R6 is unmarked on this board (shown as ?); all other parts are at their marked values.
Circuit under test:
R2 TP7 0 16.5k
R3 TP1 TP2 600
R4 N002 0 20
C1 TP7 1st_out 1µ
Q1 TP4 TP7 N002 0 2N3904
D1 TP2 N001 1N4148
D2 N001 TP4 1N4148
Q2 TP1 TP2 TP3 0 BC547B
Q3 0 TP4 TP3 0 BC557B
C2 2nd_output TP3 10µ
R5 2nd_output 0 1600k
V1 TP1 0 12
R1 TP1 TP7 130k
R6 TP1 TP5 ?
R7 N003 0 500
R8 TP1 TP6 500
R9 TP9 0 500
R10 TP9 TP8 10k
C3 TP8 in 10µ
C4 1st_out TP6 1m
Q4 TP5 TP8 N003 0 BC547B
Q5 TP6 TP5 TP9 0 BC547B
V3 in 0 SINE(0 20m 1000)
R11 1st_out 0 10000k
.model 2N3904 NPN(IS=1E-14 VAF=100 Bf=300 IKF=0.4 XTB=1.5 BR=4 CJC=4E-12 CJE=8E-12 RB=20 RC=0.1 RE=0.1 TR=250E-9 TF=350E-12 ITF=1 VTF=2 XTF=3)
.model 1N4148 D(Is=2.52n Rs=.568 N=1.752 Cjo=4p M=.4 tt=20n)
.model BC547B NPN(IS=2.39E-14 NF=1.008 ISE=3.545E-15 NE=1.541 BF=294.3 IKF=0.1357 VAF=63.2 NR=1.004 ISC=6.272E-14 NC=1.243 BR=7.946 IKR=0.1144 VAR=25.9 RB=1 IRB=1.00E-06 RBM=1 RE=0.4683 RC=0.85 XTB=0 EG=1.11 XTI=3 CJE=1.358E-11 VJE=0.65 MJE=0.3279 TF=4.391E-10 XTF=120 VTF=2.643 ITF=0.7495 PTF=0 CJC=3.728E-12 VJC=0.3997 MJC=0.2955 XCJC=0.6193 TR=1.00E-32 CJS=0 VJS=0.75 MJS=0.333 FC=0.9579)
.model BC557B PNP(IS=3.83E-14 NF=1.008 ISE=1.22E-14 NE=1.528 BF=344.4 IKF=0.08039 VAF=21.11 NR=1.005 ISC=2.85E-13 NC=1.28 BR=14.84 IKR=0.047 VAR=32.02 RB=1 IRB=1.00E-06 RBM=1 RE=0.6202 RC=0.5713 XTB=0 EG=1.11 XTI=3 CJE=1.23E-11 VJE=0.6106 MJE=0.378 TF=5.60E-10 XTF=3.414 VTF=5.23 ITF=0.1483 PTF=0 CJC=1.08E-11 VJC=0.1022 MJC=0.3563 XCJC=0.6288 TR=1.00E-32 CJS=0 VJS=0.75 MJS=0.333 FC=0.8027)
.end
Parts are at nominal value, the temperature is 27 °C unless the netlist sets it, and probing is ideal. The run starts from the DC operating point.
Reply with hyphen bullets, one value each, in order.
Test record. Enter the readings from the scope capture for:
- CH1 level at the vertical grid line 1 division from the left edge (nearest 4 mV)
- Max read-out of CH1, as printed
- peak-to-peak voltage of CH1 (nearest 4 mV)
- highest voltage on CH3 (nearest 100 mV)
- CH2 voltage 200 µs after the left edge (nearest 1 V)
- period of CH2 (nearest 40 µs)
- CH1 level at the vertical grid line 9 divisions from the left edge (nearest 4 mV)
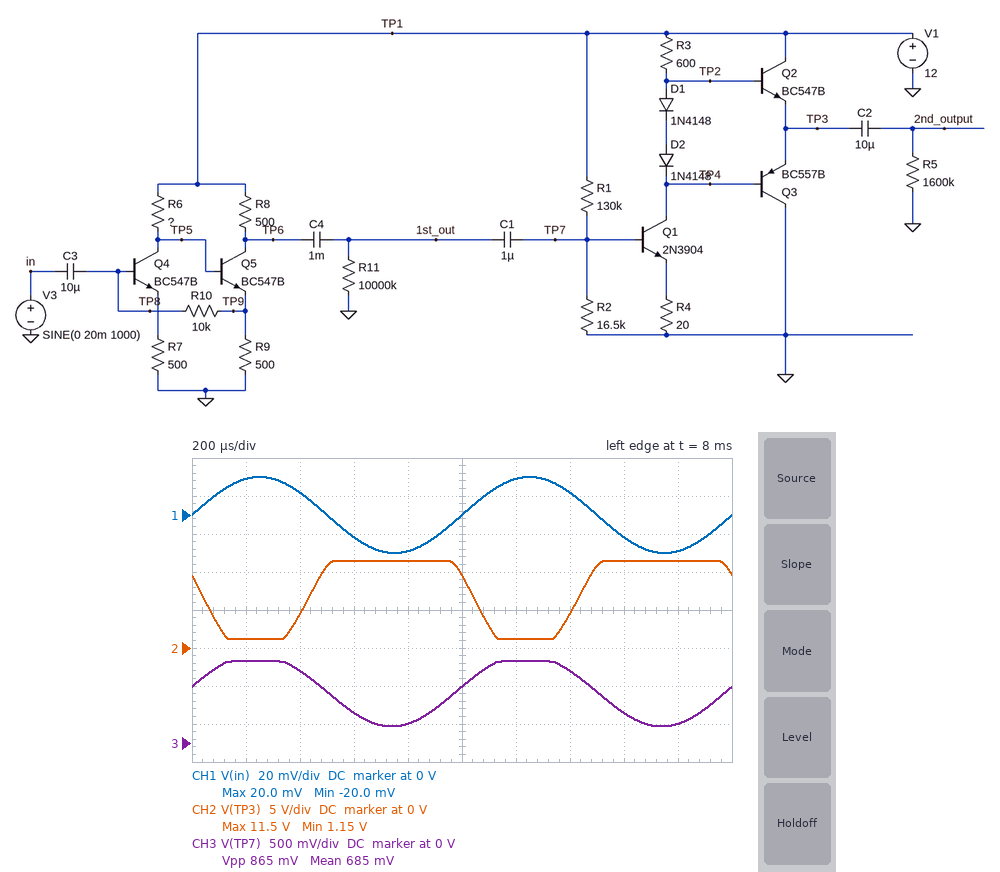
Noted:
- 20 mV
- 20.0 mV
- 40 mV
- 1.1 V
- 1 V
- 1.00 ms
- -20 mV
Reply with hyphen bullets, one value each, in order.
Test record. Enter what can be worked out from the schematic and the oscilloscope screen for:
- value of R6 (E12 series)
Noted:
- 15 kΩ
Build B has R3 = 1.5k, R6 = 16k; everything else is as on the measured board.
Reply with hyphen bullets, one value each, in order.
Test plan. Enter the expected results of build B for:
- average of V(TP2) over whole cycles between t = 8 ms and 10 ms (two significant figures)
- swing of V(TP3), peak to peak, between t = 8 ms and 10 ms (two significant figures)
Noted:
- 8.4 V
- 11 V
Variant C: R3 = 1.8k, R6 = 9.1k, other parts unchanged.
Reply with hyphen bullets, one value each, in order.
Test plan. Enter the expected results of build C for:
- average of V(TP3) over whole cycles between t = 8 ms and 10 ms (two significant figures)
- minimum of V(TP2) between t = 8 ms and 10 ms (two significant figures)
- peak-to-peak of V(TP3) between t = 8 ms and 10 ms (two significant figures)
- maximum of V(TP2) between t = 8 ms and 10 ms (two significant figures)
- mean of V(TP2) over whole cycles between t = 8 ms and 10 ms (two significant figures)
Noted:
- 7.3 V
- 1.5 V
- 11 V
- 12 V
- 7.9 V
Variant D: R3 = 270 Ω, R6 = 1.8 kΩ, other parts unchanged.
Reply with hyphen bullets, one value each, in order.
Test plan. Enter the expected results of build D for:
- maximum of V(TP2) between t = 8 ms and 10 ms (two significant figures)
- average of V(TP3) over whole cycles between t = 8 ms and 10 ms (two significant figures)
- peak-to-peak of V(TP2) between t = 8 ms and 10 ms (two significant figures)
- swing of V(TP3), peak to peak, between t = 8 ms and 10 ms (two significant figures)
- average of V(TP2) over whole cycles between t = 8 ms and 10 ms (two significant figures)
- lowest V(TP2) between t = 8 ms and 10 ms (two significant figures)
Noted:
- 10 V
- 8.7 V
- 1.5 V
- 1.6 V
- 9.4 V
- 8.6 V
